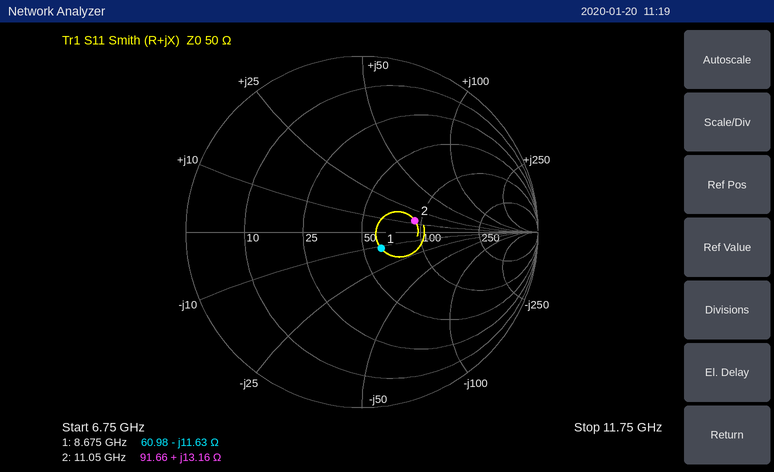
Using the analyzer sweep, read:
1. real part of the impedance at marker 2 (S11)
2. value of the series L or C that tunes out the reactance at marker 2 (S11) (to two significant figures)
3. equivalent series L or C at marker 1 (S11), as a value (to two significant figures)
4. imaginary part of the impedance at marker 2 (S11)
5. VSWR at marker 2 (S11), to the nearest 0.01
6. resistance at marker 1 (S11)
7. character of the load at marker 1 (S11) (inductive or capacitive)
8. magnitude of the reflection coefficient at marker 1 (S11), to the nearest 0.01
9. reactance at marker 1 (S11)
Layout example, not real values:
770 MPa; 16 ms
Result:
91.66 Ω; 1.1 pF; 1.6 pF; +13.16 Ω; 1.89; 60.98 Ω; capacitive; 0.14; -11.63 Ω
